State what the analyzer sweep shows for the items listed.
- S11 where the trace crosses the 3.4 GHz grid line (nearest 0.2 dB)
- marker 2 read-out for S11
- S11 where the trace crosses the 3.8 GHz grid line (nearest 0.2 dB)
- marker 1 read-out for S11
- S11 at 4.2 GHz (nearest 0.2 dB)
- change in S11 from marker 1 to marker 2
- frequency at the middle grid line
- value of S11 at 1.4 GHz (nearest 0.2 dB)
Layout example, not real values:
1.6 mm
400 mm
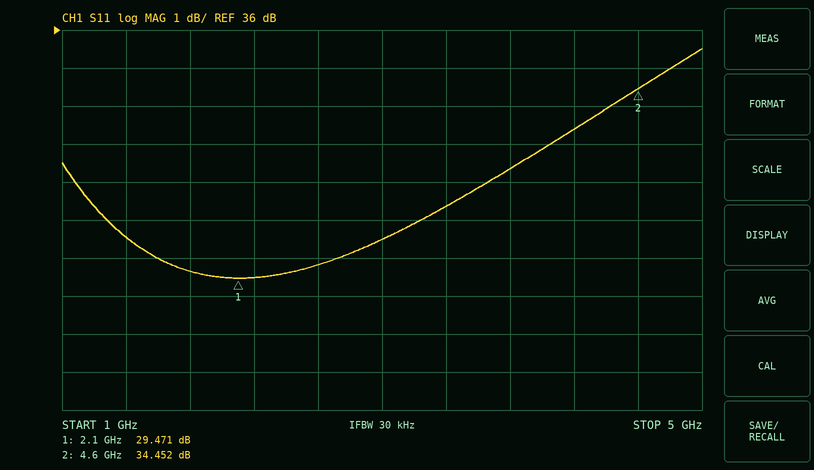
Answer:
31.4 dB
34.452 dB
32.4 dB
29.471 dB
33.4 dB
4.981 dB
3 GHz
30.6 dB
